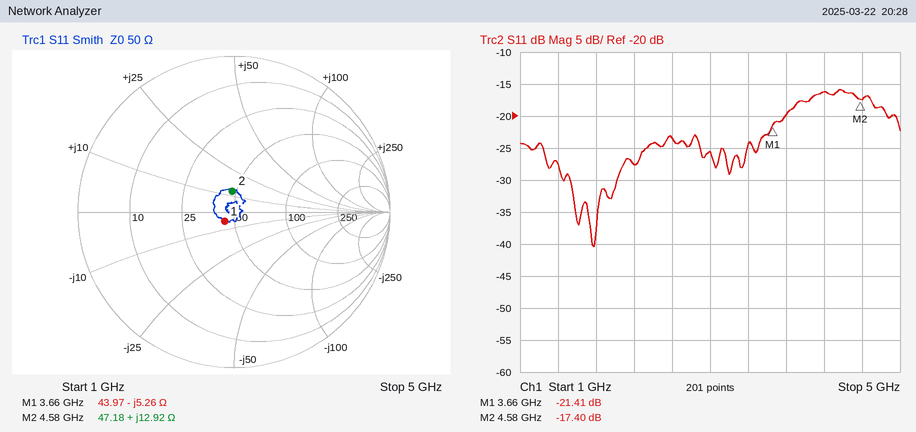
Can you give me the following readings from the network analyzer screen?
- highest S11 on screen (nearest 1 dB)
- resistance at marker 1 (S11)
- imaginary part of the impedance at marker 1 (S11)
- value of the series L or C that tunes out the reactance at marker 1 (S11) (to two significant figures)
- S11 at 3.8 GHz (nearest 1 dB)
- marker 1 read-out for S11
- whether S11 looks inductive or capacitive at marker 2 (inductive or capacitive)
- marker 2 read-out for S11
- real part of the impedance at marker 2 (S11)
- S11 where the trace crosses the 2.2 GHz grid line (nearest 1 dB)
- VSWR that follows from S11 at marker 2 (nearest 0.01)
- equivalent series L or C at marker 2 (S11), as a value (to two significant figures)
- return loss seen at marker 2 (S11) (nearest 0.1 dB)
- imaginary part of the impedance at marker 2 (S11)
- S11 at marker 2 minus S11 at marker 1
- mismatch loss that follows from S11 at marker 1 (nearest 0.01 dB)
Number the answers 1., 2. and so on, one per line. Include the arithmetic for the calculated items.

1. -16 dB
2. 43.97 Ω
3. -5.26 Ω
4. L = 5.26 Ω/(2π × 3.66 GHz) ≈ 229 pH, so 230 pH to two significant figures
5. -20 dB
6. -21.41 dB
7. inductive
8. -17.40 dB
9. 47.18 Ω
10. -28 dB
11. (1 + 0.1349)/(1 − 0.1349) ≈ 1.31
12. L = 12.92 Ω/(2π × 4.58 GHz) ≈ 449 pH, so 450 pH to two significant figures
13. 17.4 dB
14. +12.92 Ω
15. -17.4 − (-21.41) = 4.01 dB
16. −10 log10(1 − 10^(-21.41/10)) ≈ 0.03 dB
